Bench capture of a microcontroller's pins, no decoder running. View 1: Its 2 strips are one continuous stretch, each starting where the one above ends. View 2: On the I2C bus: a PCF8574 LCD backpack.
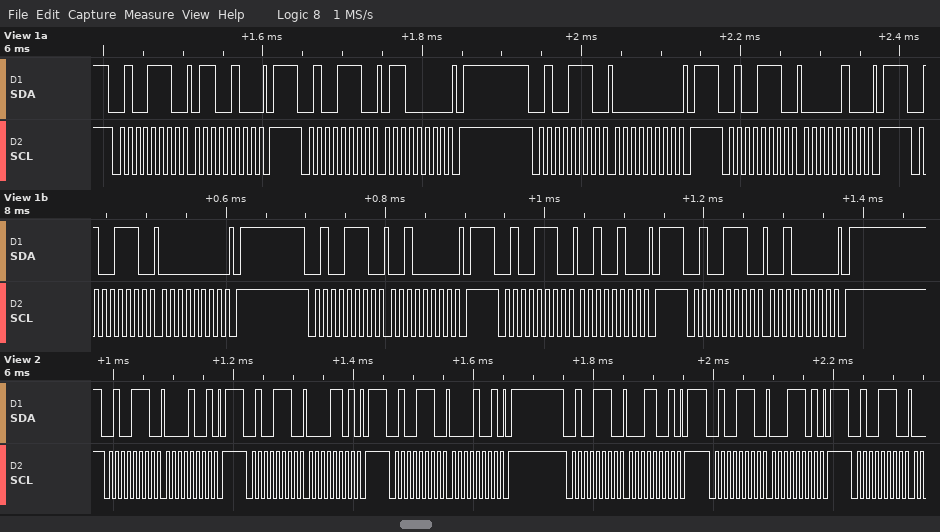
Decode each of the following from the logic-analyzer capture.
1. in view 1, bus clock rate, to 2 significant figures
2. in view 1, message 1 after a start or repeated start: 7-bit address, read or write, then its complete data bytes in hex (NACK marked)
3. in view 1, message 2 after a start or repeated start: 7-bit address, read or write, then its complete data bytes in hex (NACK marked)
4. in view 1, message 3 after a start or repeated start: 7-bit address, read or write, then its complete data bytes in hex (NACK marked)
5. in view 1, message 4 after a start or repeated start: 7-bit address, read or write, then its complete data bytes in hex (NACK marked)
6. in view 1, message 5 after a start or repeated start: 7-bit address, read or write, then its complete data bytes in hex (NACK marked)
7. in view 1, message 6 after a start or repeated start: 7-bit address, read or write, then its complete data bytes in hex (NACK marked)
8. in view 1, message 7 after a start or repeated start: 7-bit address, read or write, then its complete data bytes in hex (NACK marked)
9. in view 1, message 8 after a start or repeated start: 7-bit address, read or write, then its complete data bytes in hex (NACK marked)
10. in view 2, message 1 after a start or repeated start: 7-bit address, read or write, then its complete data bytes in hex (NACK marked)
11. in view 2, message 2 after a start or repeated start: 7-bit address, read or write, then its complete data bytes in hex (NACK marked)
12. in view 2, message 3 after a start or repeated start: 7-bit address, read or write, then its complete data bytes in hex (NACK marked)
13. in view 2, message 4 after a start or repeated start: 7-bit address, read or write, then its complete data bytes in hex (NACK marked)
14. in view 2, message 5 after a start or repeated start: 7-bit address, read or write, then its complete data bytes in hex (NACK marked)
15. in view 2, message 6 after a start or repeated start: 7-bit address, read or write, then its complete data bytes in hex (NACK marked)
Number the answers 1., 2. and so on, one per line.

1. 100 kHz
2. 0x27 write: 64
3. 0x27 write: 60
4. 0x27 write: 00
5. 0x27 write: 04
6. 0x27 write: 00
7. 0x27 write: 20
8. 0x27 write: 24
9. 0x27 write: 20
10. 0x27 write: 09
11. 0x27 write: 0D
12. 0x27 write: 09
13. 0x27 write: 19
14. 0x27 write: 1D
15. 0x27 write
